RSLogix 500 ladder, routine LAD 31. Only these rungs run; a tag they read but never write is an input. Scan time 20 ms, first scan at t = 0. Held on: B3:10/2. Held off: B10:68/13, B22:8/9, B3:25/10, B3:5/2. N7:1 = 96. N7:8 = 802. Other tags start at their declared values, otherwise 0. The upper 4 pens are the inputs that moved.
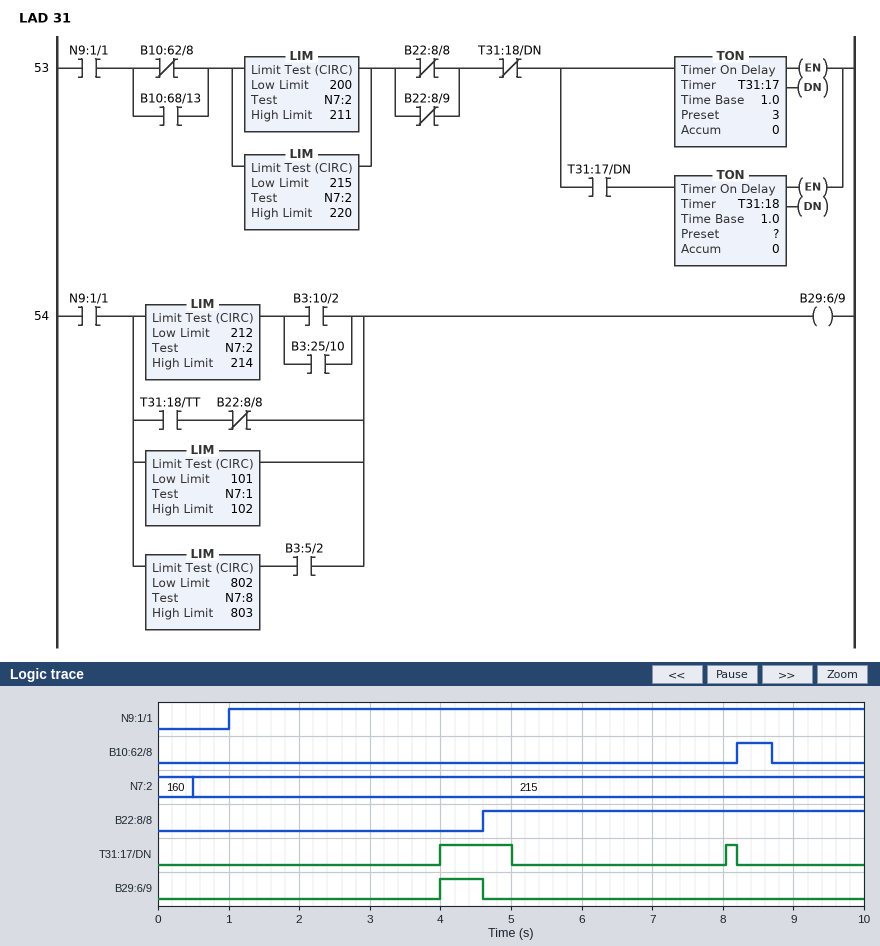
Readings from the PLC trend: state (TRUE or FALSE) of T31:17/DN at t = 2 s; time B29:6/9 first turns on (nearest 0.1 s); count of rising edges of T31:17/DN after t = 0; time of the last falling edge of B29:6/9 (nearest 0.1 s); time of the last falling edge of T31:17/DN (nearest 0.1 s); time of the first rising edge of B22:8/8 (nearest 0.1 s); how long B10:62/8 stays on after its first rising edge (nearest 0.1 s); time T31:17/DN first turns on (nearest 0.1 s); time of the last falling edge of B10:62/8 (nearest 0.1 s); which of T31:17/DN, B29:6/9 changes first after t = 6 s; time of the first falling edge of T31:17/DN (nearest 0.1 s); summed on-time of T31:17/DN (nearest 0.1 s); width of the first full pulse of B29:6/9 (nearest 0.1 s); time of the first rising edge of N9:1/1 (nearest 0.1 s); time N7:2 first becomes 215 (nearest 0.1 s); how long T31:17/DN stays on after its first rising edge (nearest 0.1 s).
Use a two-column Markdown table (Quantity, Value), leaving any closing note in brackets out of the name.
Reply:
| Quantity | Value |
|---|---|
| state (TRUE or FALSE) of T31:17/DN at t = 2 s | FALSE |
| time B29:6/9 first turns on | 4.0 s |
| count of rising edges of T31:17/DN after t = 0 | 2 |
| time of the last falling edge of B29:6/9 | 4.6 s |
| time of the last falling edge of T31:17/DN | 8.2 s |
| time of the first rising edge of B22:8/8 | 4.6 s |
| how long B10:62/8 stays on after its first rising edge | 0.5 s |
| time T31:17/DN first turns on | 4.0 s |
| time of the last falling edge of B10:62/8 | 8.7 s |
| which of T31:17/DN, B29:6/9 changes first after t = 6 s | T31:17/DN |
| time of the first falling edge of T31:17/DN | 5.0 s |
| summed on-time of T31:17/DN | 1.2 s |
| width of the first full pulse of B29:6/9 | 0.6 s |
| time of the first rising edge of N9:1/1 | 1.0 s |
| time N7:2 first becomes 215 | 0.5 s |
| how long T31:17/DN stays on after its first rising edge | 1.0 s |
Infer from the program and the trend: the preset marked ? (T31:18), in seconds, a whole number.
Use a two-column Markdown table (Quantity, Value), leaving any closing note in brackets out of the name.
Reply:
| Quantity | Value |
|---|---|
| the preset marked ? (T31:18), in seconds, a whole number | 1 s |
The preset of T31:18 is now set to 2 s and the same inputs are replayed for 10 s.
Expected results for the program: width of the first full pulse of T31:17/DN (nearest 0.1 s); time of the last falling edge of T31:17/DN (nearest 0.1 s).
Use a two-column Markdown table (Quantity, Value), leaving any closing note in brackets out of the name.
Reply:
| Quantity | Value |
|---|---|
| width of the first full pulse of T31:17/DN | 2.0 s |
| time of the last falling edge of T31:17/DN | 6.0 s |
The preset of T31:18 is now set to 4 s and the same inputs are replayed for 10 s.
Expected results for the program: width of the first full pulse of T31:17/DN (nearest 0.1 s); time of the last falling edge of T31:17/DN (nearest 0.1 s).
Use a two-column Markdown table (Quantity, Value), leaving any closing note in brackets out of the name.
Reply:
| Quantity | Value |
|---|---|
| width of the first full pulse of T31:17/DN | 4.0 s |
| time of the last falling edge of T31:17/DN | 8.0 s |
